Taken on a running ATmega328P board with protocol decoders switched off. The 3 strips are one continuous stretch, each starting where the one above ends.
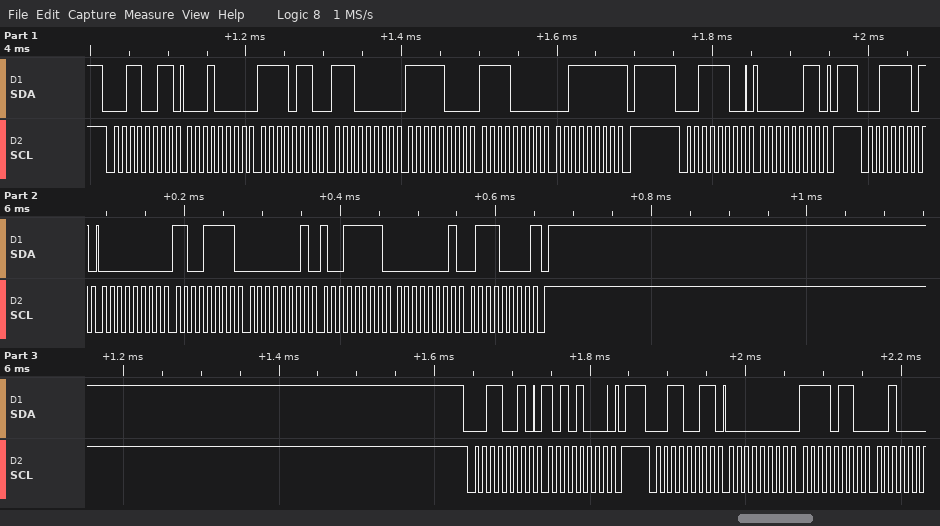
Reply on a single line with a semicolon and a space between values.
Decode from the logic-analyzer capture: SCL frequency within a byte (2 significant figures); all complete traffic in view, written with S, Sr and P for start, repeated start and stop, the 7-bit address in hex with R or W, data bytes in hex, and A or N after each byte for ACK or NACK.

100 kHz; S 19R A 10 A F6 A E0 A F8 A F0 A 3F N P S 1EW A 03 A P S 1ER A 00 A CF A 01 A 9F A 01 A 70 N P S 19W A A8 A P S 19R A 00 A F6 A
